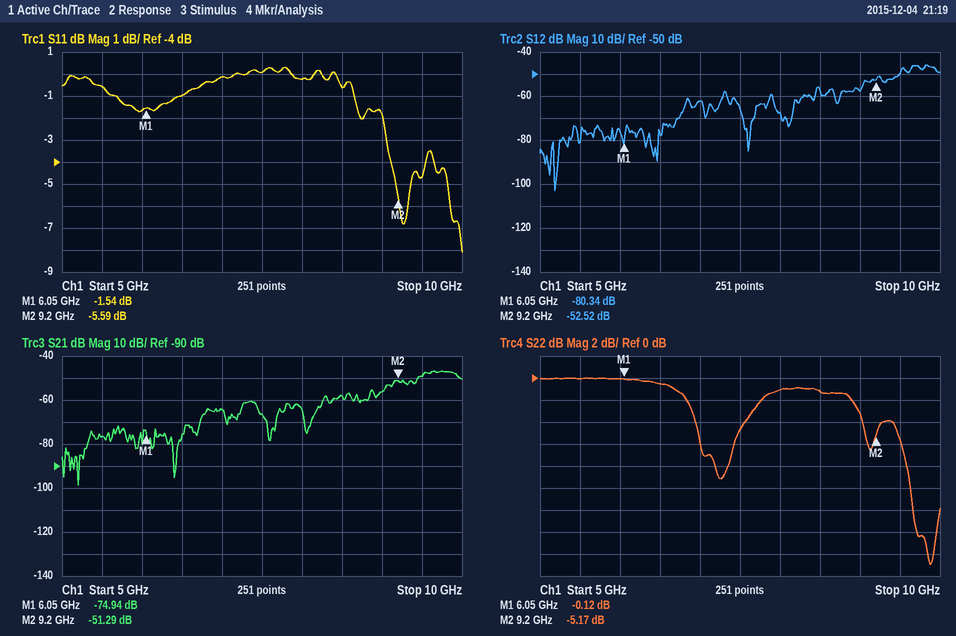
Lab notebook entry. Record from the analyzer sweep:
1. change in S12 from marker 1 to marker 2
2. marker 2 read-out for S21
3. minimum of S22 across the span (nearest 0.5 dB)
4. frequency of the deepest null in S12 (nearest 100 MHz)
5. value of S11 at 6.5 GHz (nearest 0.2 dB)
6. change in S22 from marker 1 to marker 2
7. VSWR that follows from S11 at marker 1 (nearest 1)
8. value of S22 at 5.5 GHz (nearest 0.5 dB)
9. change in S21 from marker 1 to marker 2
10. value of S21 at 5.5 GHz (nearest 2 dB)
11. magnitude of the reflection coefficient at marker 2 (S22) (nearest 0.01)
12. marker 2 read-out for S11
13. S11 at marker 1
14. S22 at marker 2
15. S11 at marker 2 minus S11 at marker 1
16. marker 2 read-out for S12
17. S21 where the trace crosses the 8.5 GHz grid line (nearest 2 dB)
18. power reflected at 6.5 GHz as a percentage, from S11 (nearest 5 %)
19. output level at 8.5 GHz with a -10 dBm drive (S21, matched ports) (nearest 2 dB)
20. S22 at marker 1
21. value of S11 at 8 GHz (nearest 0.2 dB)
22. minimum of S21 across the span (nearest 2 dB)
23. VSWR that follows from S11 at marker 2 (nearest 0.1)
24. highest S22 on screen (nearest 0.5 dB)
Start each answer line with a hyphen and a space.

- 27.82 dB
- -51.29 dB
- -17.0 dB
- 5.2 GHz
- -1.0 dB
- -5.05 dB
- 11
- 0.0 dB
- 23.65 dB
- -76 dB
- 0.55
- -5.59 dB
- -1.54 dB
- -5.17 dB
- -4.05 dB
- -52.52 dB
- -58 dB
- 80 %
- -68 dBm
- -0.12 dB
- -0.2 dB
- -98 dB
- 3.2
- 0.0 dB
